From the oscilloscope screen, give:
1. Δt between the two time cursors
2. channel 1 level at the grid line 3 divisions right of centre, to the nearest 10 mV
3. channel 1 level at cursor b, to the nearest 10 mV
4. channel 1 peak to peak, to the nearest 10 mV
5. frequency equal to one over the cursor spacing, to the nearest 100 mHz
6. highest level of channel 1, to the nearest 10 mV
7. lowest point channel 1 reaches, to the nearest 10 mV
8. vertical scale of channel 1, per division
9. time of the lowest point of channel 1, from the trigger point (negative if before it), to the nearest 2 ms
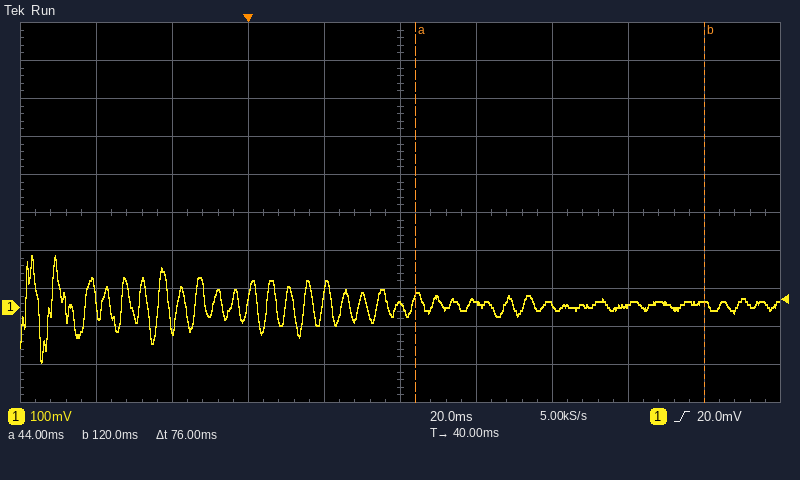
76 ms
10 mV
10 mV
280 mV
13.2 Hz
140 mV
-140 mV
100 mV
-54 ms
